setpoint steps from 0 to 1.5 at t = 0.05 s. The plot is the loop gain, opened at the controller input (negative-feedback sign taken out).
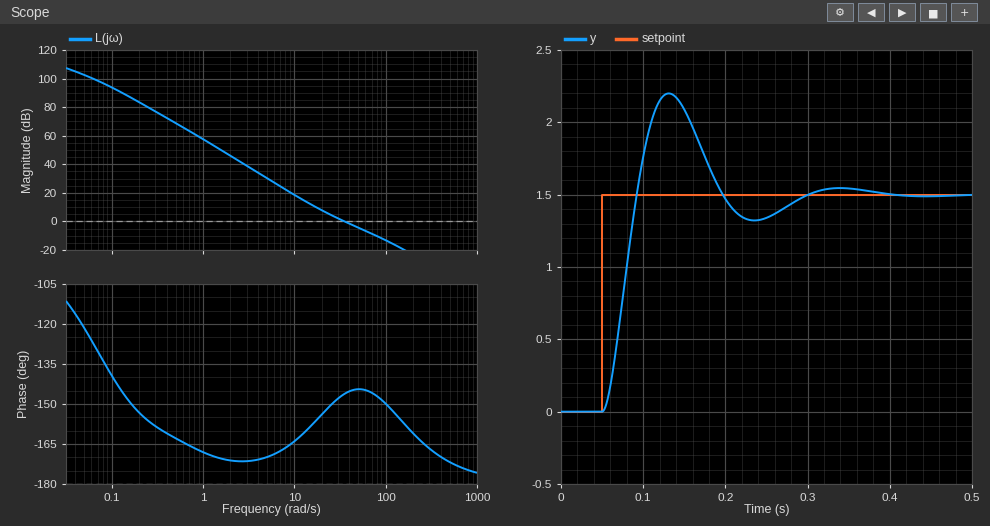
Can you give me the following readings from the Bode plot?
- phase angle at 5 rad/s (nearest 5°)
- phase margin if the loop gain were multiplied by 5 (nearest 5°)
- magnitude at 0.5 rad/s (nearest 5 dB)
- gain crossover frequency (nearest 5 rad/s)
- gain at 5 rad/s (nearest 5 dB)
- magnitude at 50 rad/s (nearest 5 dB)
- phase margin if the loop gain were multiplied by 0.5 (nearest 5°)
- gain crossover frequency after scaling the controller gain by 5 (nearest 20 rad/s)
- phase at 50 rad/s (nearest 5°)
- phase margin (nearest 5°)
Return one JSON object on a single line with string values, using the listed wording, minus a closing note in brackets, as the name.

{"phase angle at 5 rad/s": "-170°", "phase margin if the loop gain were multiplied by 5": "30°", "magnitude at 0.5 rad/s": "70 dB", "gain crossover frequency": "35 rad/s", "gain at 5 rad/s": "30 dB", "magnitude at 50 rad/s": "-5 dB", "phase margin if the loop gain were multiplied by 0.5": "30°", "gain crossover frequency after scaling the controller gain by 5": "100 rad/s", "phase at 50 rad/s": "-145°", "phase margin": "35°"}
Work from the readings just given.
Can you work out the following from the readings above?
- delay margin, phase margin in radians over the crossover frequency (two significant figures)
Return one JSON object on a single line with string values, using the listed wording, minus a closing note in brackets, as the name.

{"delay margin, phase margin in radians over the crossover frequency": "0.017 s"}
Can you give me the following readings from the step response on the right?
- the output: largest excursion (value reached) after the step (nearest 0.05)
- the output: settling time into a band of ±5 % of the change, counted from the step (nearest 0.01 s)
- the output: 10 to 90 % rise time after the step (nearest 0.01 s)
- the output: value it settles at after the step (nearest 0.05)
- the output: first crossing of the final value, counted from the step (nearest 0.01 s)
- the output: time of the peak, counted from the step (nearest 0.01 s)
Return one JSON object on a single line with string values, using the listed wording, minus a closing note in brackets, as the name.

{"the output: largest excursion (value reached) after the step": "2.20", "the output: settling time into a band of ±5 % of the change, counted from the step": "0.23 s", "the output: 10 to 90 % rise time after the step": "0.03 s", "the output: value it settles at after the step": "1.50", "the output: first crossing of the final value, counted from the step": "0.04 s", "the output: time of the peak, counted from the step": "0.08 s"}
